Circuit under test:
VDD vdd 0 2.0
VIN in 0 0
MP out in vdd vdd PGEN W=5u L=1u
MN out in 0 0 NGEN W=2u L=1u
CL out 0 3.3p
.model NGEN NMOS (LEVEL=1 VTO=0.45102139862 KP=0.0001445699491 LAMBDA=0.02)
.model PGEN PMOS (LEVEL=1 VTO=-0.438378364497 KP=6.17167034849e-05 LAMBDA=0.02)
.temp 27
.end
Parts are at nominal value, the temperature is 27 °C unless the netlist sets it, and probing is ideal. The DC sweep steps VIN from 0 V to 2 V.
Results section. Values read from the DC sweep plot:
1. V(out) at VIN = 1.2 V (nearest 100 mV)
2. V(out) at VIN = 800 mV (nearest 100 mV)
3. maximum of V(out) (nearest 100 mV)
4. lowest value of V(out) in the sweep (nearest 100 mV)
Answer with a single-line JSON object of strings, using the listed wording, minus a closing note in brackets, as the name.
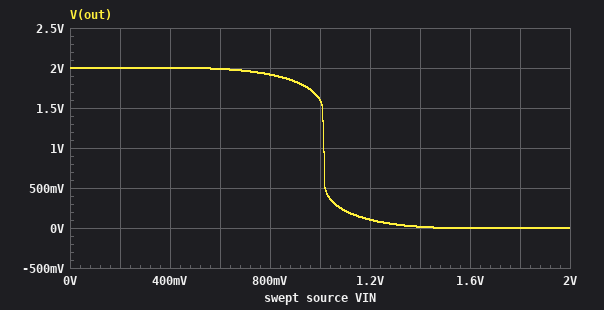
{"V(out) at VIN = 1.2 V": "100 mV", "V(out) at VIN = 800 mV": "1.9 V", "maximum of V(out)": "2.0 V", "lowest value of V(out) in the sweep": "0 V"}
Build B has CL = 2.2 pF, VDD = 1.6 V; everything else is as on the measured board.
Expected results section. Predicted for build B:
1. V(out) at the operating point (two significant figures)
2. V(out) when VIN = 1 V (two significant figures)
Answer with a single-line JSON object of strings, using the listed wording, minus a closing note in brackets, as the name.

{"V(out) at the operating point": "1.6 V", "V(out) when VIN = 1 V": "27 mV"}
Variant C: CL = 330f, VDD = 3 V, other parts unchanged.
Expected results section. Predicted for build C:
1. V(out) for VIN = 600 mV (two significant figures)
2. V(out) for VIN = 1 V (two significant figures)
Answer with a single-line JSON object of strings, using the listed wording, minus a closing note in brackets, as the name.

{"V(out) for VIN = 600 mV": "3.0 V", "V(out) for VIN = 1 V": "2.9 V"}
